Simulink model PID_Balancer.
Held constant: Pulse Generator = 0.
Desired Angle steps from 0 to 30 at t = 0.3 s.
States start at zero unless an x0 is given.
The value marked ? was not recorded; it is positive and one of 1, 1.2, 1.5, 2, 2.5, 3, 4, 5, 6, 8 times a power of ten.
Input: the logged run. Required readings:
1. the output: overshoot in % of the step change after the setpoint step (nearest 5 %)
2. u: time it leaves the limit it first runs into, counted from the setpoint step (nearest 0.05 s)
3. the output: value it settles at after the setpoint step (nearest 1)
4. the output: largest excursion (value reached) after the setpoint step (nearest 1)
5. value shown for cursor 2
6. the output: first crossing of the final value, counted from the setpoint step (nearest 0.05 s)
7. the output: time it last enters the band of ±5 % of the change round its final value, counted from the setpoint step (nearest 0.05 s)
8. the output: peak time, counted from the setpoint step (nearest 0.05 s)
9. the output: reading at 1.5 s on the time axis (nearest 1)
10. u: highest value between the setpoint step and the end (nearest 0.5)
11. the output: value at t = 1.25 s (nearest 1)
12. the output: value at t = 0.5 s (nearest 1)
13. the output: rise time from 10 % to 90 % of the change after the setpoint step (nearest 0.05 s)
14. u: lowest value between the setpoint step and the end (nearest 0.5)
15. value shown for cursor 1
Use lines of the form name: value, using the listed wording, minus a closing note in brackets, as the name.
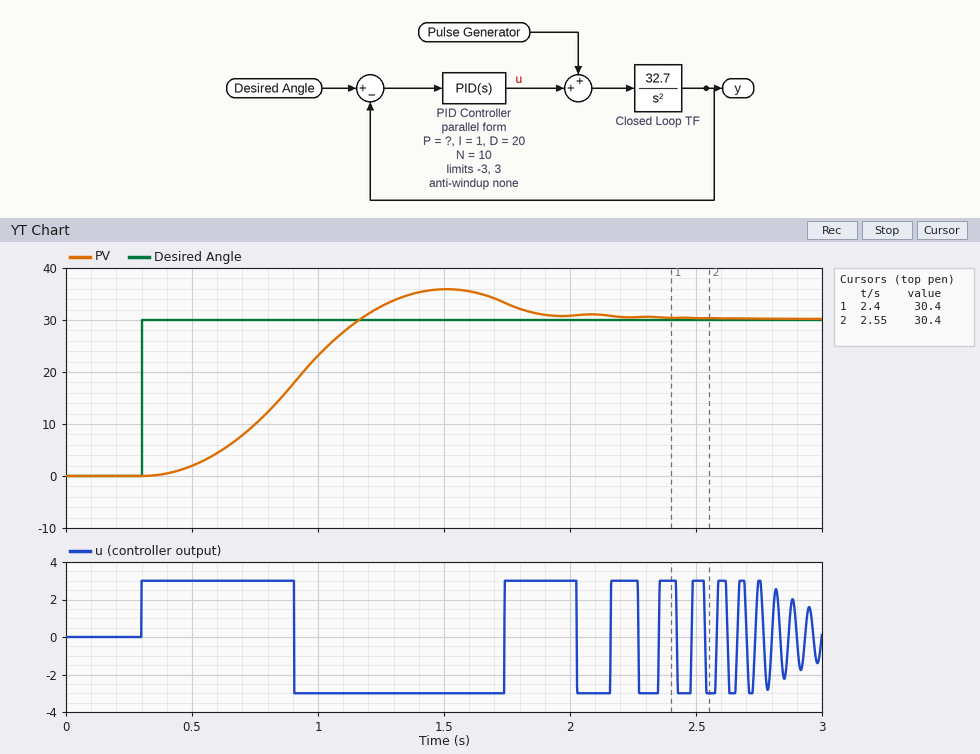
the output: overshoot in % of the step change after the setpoint step: 20 %
u: time it leaves the limit it first runs into, counted from the setpoint step: 0.60 s
the output: value it settles at after the setpoint step: 30
the output: largest excursion (value reached) after the setpoint step: 36
value shown for cursor 2: 30.4
the output: first crossing of the final value, counted from the setpoint step: 0.85 s
the output: time it last enters the band of ±5 % of the change round its final value, counted from the setpoint step: 1.55 s
the output: peak time, counted from the setpoint step: 1.20 s
the output: reading at 1.5 s on the time axis: 36
u: highest value between the setpoint step and the end: 3.0
the output: value at t = 1.25 s: 33
the output: value at t = 0.5 s: 2
the output: rise time from 10 % to 90 % of the change after the setpoint step: 0.55 s
u: lowest value between the setpoint step and the end: -3.0
value shown for cursor 1: 30.4
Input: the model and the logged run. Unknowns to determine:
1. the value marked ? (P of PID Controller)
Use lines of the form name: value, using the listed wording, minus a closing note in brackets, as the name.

the value marked ?: 80
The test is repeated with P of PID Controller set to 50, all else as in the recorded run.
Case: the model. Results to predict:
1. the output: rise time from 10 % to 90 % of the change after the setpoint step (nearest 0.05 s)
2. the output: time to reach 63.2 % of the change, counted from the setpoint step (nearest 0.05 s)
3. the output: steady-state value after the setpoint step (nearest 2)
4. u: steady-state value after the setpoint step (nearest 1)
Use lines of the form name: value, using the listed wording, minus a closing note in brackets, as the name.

the output: rise time from 10 % to 90 % of the change after the setpoint step: 0.70 s
the output: time to reach 63.2 % of the change, counted from the setpoint step: 0.65 s
the output: steady-state value after the setpoint step: 30
u: steady-state value after the setpoint step: 0
